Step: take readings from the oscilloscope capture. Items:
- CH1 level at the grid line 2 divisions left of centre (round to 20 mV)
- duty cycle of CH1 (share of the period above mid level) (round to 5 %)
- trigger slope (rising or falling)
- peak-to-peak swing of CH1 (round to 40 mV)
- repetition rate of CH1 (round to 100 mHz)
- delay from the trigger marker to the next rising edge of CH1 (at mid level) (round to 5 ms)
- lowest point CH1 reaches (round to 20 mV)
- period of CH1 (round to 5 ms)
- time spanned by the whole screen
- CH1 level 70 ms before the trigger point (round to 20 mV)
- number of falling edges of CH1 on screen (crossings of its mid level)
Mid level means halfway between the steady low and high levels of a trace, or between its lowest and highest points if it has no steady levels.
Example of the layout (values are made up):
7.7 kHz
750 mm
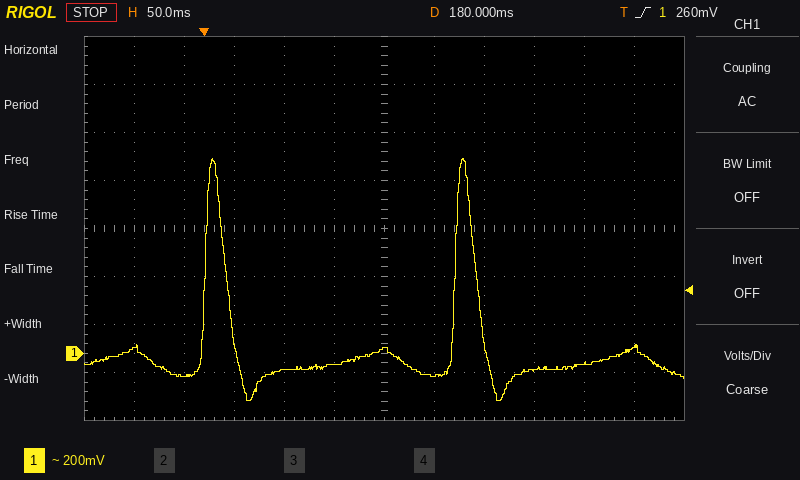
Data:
-60 mV
10 %
rising
1.00 V
4.0 Hz
250 ms
-200 mV
250 ms
600 ms
20 mV
2
